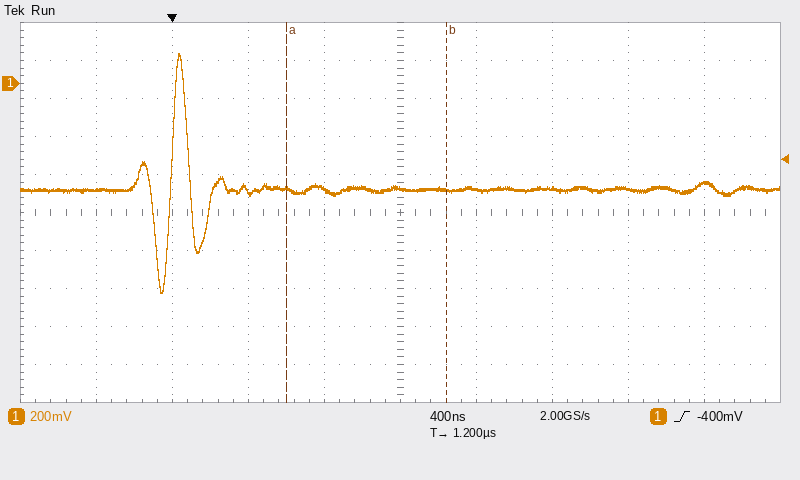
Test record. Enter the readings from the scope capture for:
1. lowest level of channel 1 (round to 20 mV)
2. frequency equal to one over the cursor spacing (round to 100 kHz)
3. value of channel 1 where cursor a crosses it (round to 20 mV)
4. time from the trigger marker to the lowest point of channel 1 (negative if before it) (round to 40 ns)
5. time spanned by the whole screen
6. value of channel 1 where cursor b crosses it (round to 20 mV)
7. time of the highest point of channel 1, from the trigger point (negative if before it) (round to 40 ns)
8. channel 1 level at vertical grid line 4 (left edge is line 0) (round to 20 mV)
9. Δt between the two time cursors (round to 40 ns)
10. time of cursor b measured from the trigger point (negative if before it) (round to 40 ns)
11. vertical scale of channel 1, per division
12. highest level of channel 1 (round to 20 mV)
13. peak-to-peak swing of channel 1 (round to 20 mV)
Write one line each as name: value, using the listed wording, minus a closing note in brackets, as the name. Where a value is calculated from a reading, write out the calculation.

lowest level of channel 1: -1.10 V
frequency equal to one over the cursor spacing: 1 / 840 ns ≈ 1.2 MHz
value of channel 1 where cursor a crosses it: -560 mV
time from the trigger marker to the lowest point of channel 1 (negative if before it): -40 ns
time spanned by the whole screen: 4 µs
value of channel 1 where cursor b crosses it: -560 mV
time of the highest point of channel 1, from the trigger point (negative if before it): +40 ns
channel 1 level at vertical grid line 4 (left edge is line 0): -560 mV
Δt between the two time cursors: 840 ns
time of cursor b measured from the trigger point (negative if before it): +1.44 µs
vertical scale of channel 1, per division: 200 mV
highest level of channel 1: 160 mV
peak-to-peak swing of channel 1: 160 mV − (-1.10 V) = 1.26 V
